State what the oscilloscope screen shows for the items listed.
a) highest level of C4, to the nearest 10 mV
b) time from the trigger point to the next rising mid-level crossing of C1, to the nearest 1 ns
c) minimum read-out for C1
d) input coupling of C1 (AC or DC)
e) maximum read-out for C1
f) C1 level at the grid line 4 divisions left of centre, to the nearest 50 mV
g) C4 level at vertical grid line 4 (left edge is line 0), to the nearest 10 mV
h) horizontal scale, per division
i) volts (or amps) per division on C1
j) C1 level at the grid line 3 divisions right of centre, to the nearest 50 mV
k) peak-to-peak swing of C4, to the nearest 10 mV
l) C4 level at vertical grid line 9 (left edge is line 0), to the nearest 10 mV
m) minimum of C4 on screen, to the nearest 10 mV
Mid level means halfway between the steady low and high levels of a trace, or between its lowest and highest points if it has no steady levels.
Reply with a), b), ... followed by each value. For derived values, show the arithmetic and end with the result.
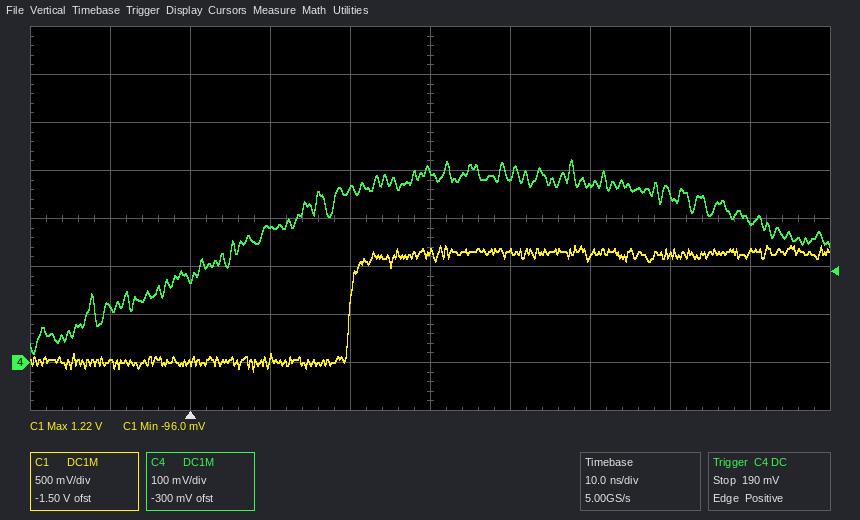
a) 420 mV
b) 20 ns
c) -96.0 mV
d) DC
e) 1.22 V
f) 0 mV
g) 360 mV
h) 10 ns
i) 500 mV
j) 1.15 V
k) 420 mV − (20 mV) = 400 mV
l) 300 mV
m) 20 mV
